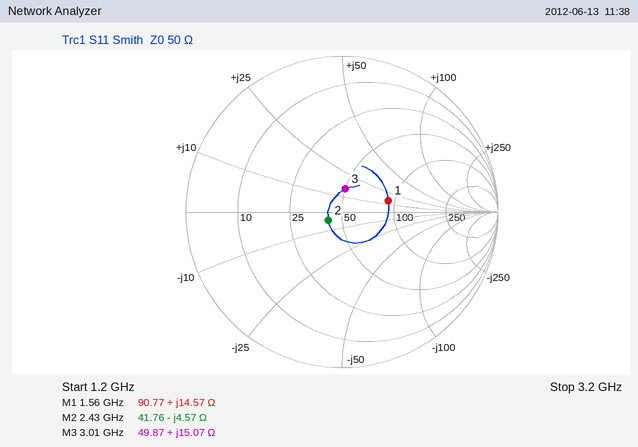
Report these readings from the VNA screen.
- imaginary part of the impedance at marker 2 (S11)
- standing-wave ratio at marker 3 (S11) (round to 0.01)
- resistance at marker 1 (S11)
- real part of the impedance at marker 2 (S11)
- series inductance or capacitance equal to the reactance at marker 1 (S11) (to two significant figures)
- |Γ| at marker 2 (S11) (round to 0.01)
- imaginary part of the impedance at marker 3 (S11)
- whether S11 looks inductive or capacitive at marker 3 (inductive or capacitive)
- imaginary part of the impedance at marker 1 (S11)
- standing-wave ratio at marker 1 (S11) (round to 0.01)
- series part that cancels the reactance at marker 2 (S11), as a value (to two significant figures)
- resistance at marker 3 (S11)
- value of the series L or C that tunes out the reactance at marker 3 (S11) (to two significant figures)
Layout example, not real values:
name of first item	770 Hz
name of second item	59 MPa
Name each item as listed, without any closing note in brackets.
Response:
imaginary part of the impedance at marker 2	-4.57 Ω
standing-wave ratio at marker 3 (S11)	1.35
resistance at marker 1	90.77 Ω
real part of the impedance at marker 2	41.76 Ω
series inductance or capacitance equal to the reactance at marker 1 (S11)	1.5 nH
|Γ| at marker 2 (S11)	0.10
imaginary part of the impedance at marker 3	+15.07 Ω
whether S11 looks inductive or capacitive at marker 3	inductive
imaginary part of the impedance at marker 1	+14.57 Ω
standing-wave ratio at marker 1 (S11)	1.88
series part that cancels the reactance at marker 2 (S11), as a value	300 pH
resistance at marker 3	49.87 Ω
value of the series L or C that tunes out the reactance at marker 3 (S11)	3.5 pF
